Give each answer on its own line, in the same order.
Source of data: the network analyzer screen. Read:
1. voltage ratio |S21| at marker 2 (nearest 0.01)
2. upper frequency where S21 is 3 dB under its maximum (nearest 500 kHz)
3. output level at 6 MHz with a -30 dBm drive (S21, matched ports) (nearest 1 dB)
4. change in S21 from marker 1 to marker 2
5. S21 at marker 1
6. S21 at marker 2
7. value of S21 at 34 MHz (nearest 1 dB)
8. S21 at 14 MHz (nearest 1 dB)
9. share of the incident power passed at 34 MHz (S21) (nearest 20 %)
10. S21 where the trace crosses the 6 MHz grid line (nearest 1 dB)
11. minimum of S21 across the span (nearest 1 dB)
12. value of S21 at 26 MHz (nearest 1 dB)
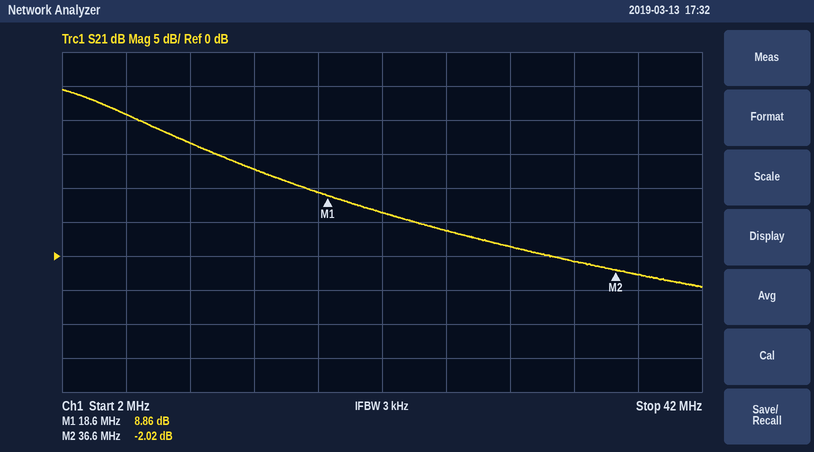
0.79
5.5 MHz
-9 dBm
-10.88 dB
8.86 dB
-2.02 dB
-1 dB
13 dB
80 %
21 dB
-5 dB
4 dB
